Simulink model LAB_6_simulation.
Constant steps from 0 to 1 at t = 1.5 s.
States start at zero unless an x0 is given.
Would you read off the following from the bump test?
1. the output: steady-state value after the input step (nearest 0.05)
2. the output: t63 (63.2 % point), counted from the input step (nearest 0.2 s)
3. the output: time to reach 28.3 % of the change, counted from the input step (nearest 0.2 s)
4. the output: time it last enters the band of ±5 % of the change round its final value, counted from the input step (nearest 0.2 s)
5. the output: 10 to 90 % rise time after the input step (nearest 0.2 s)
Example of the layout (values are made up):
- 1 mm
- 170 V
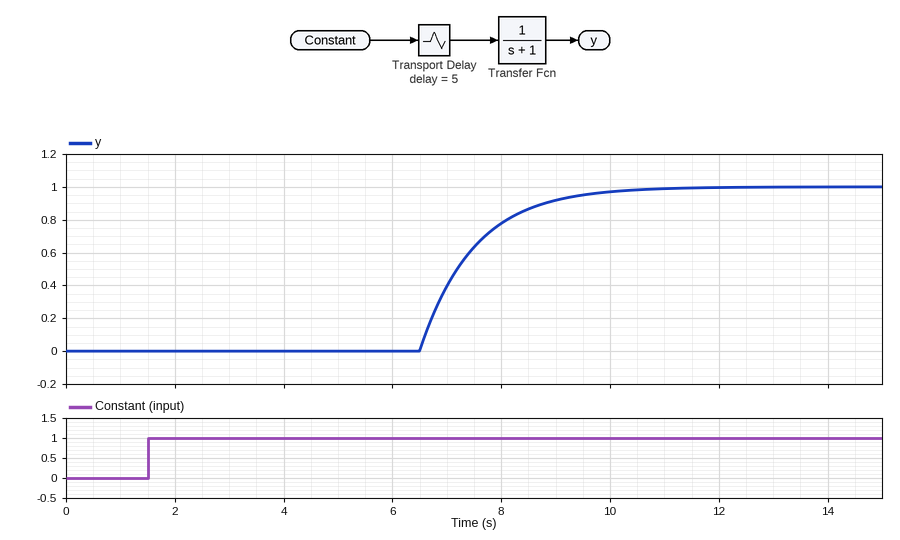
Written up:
- 1.00
- 6.0 s
- 5.4 s
- 8.0 s
- 2.2 s
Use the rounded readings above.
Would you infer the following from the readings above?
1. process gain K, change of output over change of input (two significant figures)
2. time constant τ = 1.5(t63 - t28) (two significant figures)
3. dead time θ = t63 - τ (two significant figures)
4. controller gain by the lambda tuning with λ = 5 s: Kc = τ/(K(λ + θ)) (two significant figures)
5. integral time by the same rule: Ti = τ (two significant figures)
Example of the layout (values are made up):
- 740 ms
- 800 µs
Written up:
- 1.0
- 0.90 s
- 5.1 s
- 0.089
- 0.90 s
